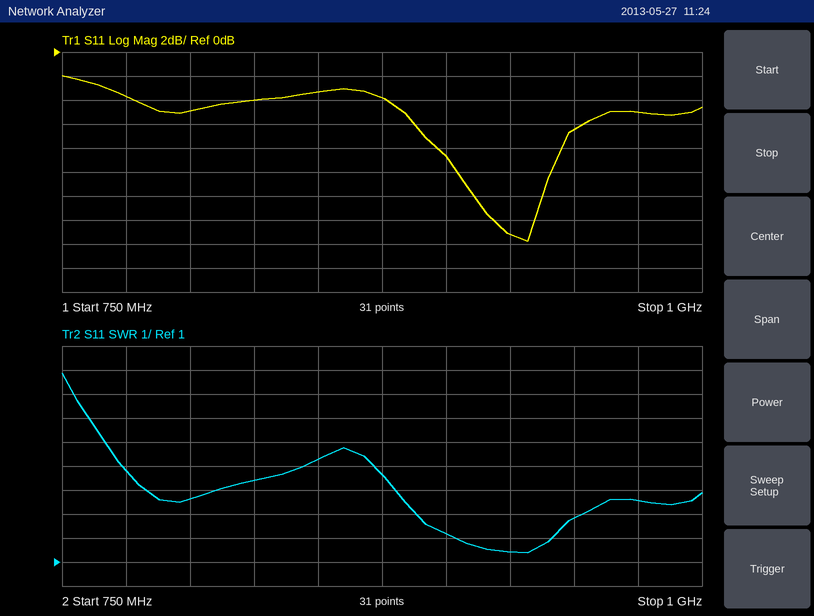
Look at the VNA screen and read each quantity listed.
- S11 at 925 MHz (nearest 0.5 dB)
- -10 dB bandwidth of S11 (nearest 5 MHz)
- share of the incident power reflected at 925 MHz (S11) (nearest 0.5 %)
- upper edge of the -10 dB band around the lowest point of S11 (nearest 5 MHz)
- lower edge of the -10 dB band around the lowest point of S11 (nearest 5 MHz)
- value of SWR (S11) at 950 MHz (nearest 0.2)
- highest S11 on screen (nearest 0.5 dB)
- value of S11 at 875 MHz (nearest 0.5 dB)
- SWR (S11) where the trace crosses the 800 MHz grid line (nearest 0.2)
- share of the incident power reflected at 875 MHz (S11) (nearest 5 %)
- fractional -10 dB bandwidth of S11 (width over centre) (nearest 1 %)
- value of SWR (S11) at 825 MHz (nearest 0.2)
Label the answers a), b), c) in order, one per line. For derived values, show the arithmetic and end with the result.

a) -15.0 dB
b) 940 MHz − 905 MHz = 35 MHz
c) 10^(-15/10) ≈ 3.16 %, so 3.0 % to the nearest 0.5 %
d) 940 MHz
e) 905 MHz
f) 2.8
g) -2.0 dB
h) -4.0 dB
i) 3.6
j) 10^(-4/10) ≈ 40 %
k) 35 MHz / 922.5 MHz ≈ 4 %
l) 4.4
